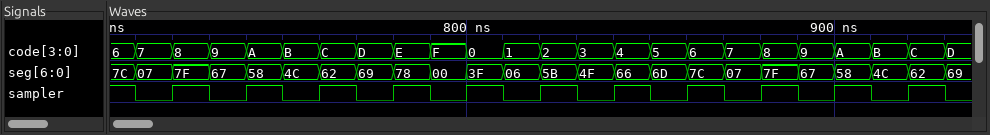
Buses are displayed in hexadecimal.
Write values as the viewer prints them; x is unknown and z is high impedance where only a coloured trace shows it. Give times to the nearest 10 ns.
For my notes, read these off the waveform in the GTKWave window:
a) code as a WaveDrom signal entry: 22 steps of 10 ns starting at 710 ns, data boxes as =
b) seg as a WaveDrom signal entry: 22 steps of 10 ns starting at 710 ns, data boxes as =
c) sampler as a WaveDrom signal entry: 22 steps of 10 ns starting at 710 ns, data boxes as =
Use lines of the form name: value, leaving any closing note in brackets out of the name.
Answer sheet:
code as a WaveDrom signal entry: 22 steps of 10 ns starting at 710 ns, data boxes as =: {name: 'code', wave: '======================', data: '7 8 9 A B C D E F 0 1 2 3 4 5 6 7 8 9 A B C'}
seg as a WaveDrom signal entry: 22 steps of 10 ns starting at 710 ns, data boxes as =: {name: 'seg', wave: '======================', data: '07 7F 67 58 4C 62 69 78 00 3F 06 5B 4F 66 6D 7C 07 7F 67 58 4C 62'}
sampler as a WaveDrom signal entry: 22 steps of 10 ns starting at 710 ns, data boxes as =: {name: 'sampler', wave: '0101010101010101010101'}
